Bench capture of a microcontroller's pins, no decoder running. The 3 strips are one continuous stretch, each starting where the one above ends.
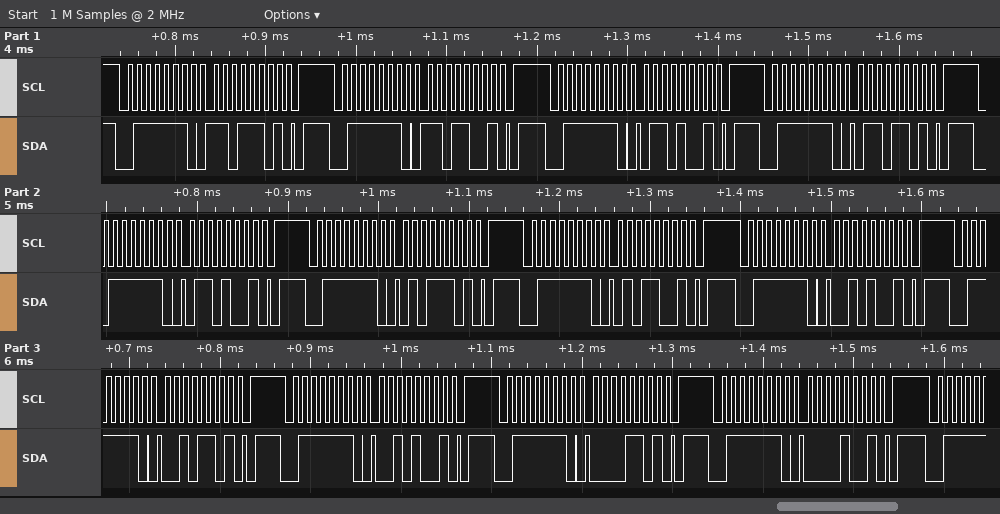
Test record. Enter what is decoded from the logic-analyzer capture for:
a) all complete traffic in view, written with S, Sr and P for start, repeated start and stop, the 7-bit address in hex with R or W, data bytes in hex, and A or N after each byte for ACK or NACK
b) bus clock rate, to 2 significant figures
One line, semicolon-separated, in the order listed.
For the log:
S 3FW A DD A P S 3FW A D9 A P S 3FW A 69 A P S 3FW A 6D A P S 3FW A 69 A P S 3FW A 5D A P S 3FW A 59 A P S 3FW A 29 A P S 3FW A 2D A P S 3FW A 29 A P S 3FW A 0D A P S 3FW A 09 A P; 100 kHz
